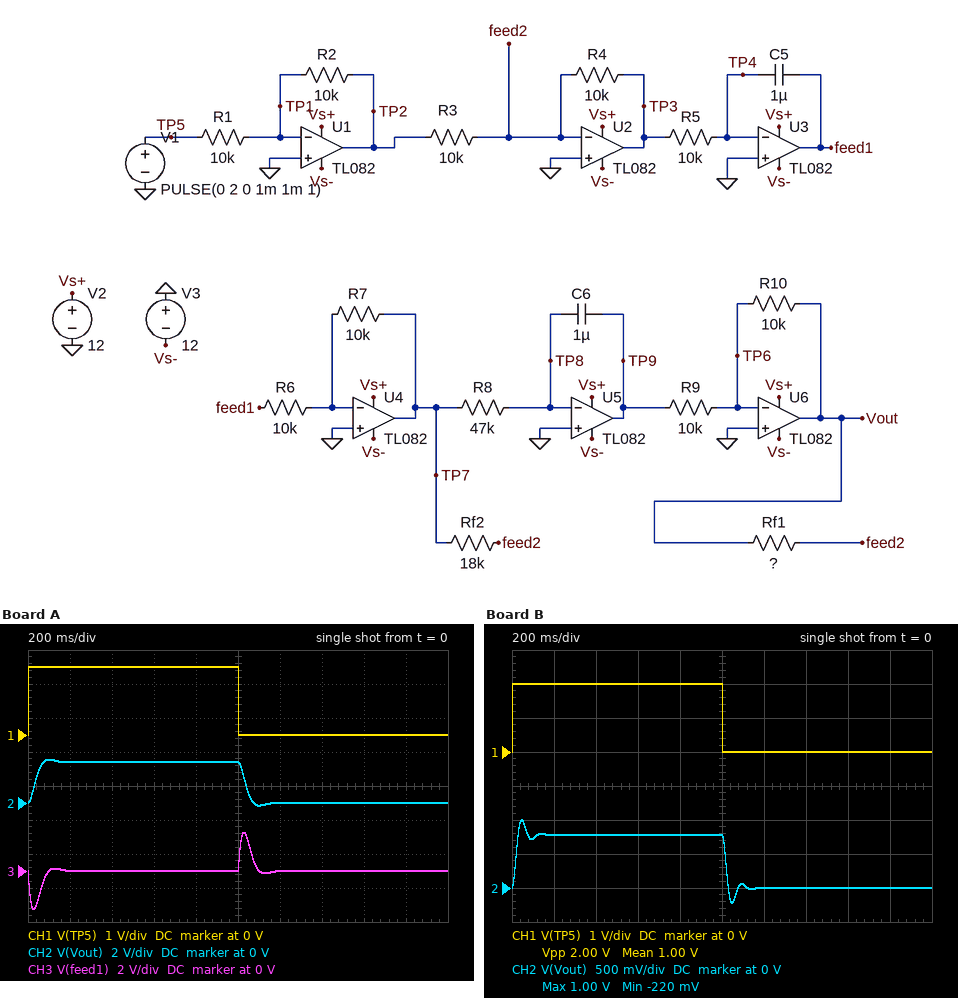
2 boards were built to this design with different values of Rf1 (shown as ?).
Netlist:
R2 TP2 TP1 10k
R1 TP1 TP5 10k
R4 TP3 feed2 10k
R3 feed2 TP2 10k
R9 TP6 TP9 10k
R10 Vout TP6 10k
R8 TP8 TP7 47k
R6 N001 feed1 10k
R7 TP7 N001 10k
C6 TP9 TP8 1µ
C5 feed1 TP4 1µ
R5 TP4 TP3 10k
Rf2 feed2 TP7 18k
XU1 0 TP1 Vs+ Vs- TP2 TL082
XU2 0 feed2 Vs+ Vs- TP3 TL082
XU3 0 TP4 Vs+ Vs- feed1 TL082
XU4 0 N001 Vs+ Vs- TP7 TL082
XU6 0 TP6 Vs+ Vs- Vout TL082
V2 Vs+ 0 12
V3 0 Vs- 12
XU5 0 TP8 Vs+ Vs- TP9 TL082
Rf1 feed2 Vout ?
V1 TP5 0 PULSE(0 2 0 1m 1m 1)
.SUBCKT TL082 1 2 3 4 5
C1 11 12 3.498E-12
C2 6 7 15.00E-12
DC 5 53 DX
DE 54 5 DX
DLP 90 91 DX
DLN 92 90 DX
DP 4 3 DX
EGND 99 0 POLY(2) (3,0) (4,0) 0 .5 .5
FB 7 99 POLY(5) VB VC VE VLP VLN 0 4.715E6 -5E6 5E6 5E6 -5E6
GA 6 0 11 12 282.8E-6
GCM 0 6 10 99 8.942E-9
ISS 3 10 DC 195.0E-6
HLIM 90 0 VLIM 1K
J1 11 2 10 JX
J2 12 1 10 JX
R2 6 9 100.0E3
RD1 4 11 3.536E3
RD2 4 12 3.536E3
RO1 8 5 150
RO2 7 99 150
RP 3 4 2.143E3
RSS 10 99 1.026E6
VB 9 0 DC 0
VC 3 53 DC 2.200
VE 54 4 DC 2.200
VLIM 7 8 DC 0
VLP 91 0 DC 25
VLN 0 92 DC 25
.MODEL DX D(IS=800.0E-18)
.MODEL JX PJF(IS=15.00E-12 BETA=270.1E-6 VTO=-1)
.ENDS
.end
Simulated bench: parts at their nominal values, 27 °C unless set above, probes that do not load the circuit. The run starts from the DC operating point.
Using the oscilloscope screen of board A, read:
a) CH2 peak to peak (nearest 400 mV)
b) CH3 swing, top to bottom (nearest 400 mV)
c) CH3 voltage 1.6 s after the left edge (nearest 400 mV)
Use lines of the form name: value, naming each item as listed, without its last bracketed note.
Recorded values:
CH2 peak to peak: 2.8 V
CH3 swing, top to bottom: 4.4 V
CH3 voltage 1.6 s after the left edge: 0 V
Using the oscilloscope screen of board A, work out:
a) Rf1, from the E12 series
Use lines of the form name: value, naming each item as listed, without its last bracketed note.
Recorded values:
Rf1, from the E12 series: 12 kΩ
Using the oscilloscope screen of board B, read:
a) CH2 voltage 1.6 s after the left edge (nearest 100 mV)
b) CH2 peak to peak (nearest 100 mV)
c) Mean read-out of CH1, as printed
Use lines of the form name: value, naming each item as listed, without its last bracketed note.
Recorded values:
CH2 voltage 1.6 s after the left edge: 0 V
CH2 peak to peak: 1.2 V
Mean read-out of CH1, as printed: 1.00 V
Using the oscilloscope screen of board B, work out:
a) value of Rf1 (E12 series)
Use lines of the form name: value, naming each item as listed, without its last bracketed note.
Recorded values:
value of Rf1: 3.9 kΩ
